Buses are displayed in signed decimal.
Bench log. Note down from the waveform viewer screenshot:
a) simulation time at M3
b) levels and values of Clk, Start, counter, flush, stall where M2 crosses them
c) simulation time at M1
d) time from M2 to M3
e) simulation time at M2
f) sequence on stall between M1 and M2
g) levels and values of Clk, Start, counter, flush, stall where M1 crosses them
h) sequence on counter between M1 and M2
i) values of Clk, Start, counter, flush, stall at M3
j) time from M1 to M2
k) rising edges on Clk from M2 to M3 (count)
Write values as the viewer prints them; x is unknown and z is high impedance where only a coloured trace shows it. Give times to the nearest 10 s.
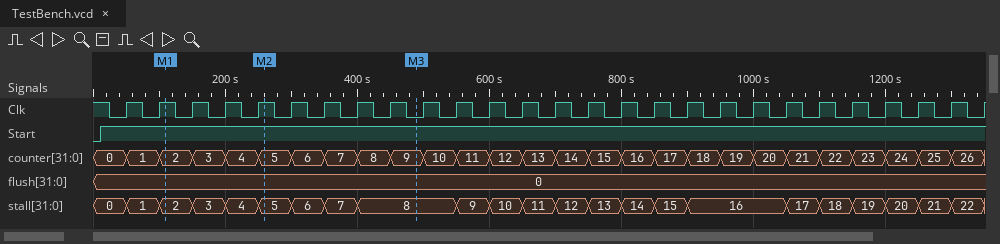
490 s
Clk=1, Start=1, counter=5, flush=0, stall=5
110 s
230 s
260 s
2, 3, 4, 5
Clk=1, Start=1, counter=2, flush=0, stall=2
2, 3, 4, 5
Clk=0, Start=1, counter=9, flush=0, stall=8
150 s
4
